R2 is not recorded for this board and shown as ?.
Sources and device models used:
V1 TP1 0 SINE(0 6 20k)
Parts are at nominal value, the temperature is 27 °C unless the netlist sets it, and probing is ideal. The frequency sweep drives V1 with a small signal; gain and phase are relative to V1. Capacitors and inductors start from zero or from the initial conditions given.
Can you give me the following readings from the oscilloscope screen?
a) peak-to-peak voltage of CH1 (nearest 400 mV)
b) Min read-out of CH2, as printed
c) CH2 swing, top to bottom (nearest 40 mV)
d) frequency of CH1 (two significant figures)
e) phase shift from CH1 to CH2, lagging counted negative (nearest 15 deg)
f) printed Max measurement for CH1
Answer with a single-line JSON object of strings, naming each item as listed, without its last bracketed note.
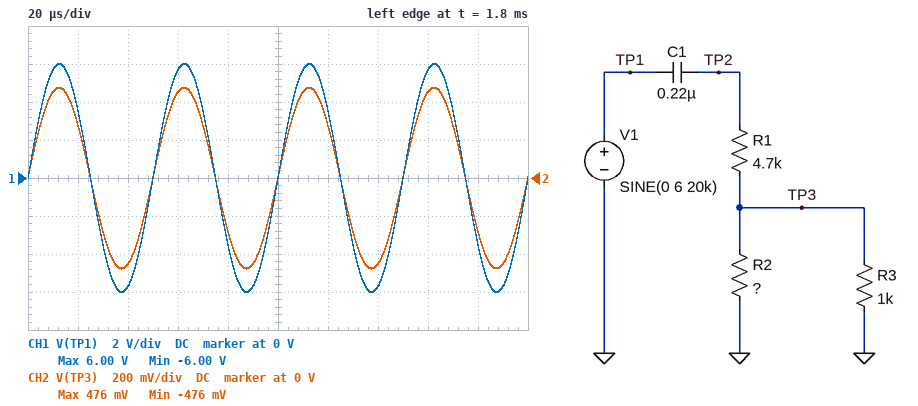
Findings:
{"peak-to-peak voltage of CH1": "12.0 V", "Min read-out of CH2, as printed": "-476 mV", "CH2 swing, top to bottom": "960 mV", "frequency of CH1": "20 kHz", "phase shift from CH1 to CH2, lagging counted negative": "0 deg", "printed Max measurement for CH1": "6.00 V"}
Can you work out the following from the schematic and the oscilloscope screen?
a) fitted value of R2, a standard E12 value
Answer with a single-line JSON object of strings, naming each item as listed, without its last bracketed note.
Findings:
{"fitted value of R2, a standard E12 value": "680 Ω"}
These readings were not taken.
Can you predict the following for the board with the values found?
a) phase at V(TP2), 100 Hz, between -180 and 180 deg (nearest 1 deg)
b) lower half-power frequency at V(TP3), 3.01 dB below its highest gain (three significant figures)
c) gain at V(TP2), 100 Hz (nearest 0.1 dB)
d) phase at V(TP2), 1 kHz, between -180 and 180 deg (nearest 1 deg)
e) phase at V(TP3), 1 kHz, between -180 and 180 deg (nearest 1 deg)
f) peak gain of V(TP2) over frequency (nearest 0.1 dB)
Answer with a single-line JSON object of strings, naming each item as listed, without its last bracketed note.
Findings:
{"phase at V(TP2), 100 Hz, between -180 and 180 deg": "55 deg", "lower half-power frequency at V(TP3), 3.01 dB below its highest gain": "142 Hz", "gain at V(TP2), 100 Hz": "-4.8 dB", "phase at V(TP2), 1 kHz, between -180 and 180 deg": "8 deg", "phase at V(TP3), 1 kHz, between -180 and 180 deg": "8 deg", "peak gain of V(TP2) over frequency": "0 dB"}
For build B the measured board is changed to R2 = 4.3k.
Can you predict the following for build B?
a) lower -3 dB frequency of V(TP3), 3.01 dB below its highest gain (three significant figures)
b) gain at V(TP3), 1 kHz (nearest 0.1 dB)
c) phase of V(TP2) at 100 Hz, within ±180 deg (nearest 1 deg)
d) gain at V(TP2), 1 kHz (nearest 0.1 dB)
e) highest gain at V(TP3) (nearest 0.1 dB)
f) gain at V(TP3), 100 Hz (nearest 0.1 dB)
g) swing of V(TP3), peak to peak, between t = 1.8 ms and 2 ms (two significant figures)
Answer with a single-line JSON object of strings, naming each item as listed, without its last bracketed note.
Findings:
{"lower -3 dB frequency of V(TP3), 3.01 dB below its highest gain": "131 Hz", "gain at V(TP3), 1 kHz": "-16.7 dB", "phase of V(TP2) at 100 Hz, within ±180 deg": "53 deg", "gain at V(TP2), 1 kHz": "-0.1 dB", "highest gain at V(TP3)": "-16.6 dB", "gain at V(TP3), 100 Hz": "-21.0 dB", "swing of V(TP3), peak to peak, between t = 1.8 ms and 2 ms": "1.8 V"}
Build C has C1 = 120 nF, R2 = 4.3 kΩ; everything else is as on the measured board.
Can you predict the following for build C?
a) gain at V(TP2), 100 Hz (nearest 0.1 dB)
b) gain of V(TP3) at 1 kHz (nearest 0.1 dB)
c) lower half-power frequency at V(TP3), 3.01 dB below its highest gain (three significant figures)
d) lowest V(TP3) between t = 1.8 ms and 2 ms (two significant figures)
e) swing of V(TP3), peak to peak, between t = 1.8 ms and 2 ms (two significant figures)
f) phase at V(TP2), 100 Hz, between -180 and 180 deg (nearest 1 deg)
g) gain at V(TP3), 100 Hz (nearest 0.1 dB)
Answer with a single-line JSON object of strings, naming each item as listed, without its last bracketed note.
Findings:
{"gain at V(TP2), 100 Hz": "-8.3 dB", "gain of V(TP3) at 1 kHz": "-16.9 dB", "lower half-power frequency at V(TP3), 3.01 dB below its highest gain": "241 Hz", "lowest V(TP3) between t = 1.8 ms and 2 ms": "-880 mV", "swing of V(TP3), peak to peak, between t = 1.8 ms and 2 ms": "1.8 V", "phase at V(TP2), 100 Hz, between -180 and 180 deg": "67 deg", "gain at V(TP3), 100 Hz": "-25.0 dB"}
